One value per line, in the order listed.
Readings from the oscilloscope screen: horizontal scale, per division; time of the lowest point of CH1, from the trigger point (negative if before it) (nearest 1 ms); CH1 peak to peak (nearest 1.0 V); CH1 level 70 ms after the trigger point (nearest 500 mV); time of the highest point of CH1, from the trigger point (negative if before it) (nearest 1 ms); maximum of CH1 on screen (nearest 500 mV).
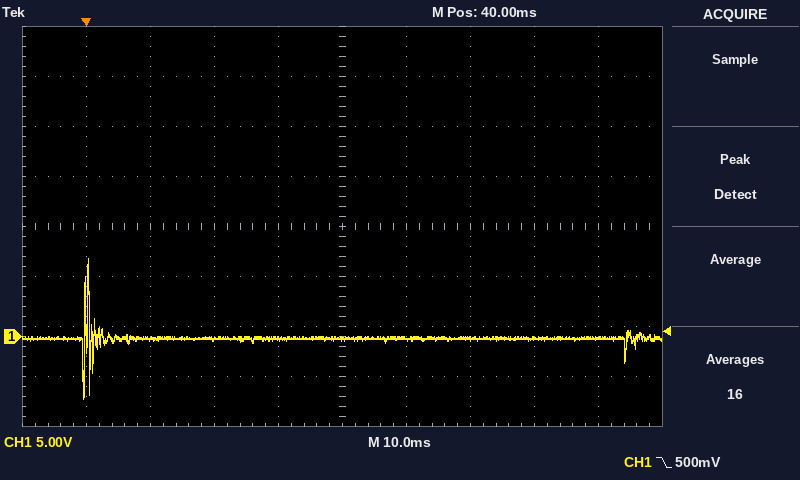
10 ms
0 ms
14.0 V
0.0 V
0 ms
8.0 V
